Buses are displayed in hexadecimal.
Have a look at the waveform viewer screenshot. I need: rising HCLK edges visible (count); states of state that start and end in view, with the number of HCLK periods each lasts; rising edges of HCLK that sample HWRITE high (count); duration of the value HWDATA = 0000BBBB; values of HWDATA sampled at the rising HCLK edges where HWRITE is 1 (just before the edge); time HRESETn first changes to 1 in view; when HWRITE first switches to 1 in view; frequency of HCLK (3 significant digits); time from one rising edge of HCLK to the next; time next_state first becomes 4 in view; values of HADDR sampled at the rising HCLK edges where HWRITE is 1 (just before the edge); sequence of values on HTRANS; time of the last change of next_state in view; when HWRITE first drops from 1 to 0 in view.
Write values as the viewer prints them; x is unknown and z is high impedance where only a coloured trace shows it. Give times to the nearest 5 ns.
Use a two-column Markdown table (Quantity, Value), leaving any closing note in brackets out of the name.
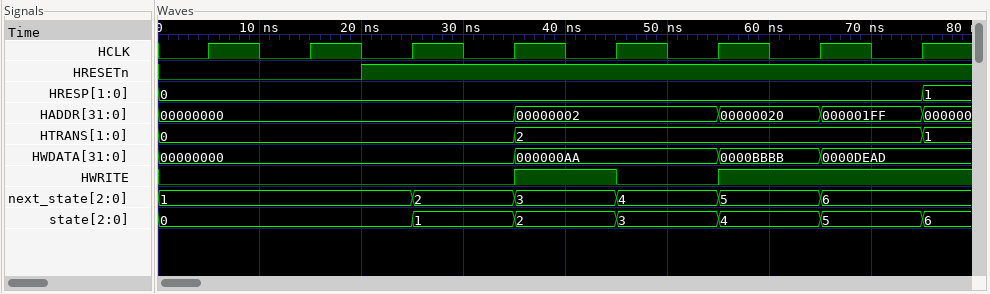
| Quantity | Value |
|---|---|
| rising HCLK edges visible | 8 |
| states of state that start and end in view, with the number of HCLK periods each lasts | 1: 1, 2: 1, 3: 1, 4: 1, 5: 1 |
| rising edges of HCLK that sample HWRITE high | 3 |
| duration of the value HWDATA = 0000BBBB | 10 ns |
| values of HWDATA sampled at the rising HCLK edges where HWRITE is 1 | 000000AA, 0000BBBB, 0000DEAD |
| time HRESETn first changes to 1 in view | 20 ns |
| when HWRITE first switches to 1 in view | 35 ns |
| frequency of HCLK | 100 MHz |
| time from one rising edge of HCLK to the next | 10 ns |
| time next_state first becomes 4 in view | 45 ns |
| values of HADDR sampled at the rising HCLK edges where HWRITE is 1 | 00000002, 00000020, 000001FF |
| sequence of values on HTRANS | 0, 2, 1 |
| time of the last change of next_state in view | 65 ns |
| when HWRITE first drops from 1 to 0 in view | 45 ns |
